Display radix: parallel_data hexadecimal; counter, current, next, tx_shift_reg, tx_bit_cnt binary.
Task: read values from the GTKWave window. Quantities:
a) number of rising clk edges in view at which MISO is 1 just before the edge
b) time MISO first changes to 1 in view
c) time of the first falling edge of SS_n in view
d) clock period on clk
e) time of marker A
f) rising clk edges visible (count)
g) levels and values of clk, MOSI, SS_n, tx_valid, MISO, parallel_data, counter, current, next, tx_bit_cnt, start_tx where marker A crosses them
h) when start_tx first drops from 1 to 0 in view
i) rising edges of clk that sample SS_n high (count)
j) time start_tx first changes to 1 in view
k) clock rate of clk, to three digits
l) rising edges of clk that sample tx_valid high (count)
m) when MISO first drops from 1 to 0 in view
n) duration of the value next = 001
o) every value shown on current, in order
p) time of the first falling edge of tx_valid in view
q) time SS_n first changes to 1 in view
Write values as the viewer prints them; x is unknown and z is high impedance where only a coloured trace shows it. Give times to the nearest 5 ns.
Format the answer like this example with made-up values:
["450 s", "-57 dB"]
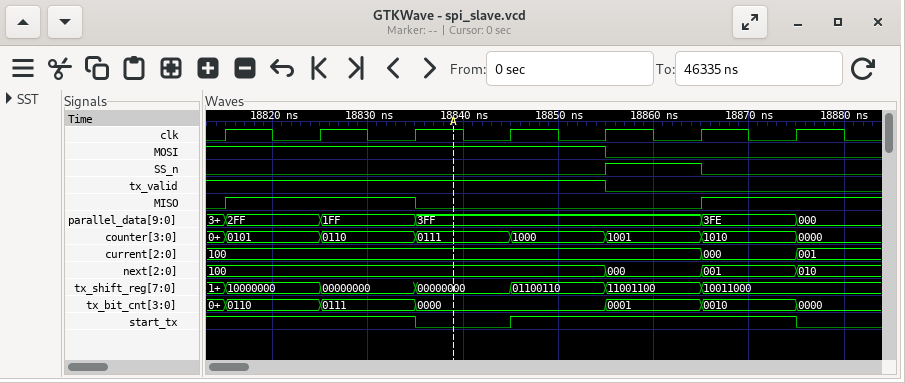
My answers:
["3", "18815 ns", "18865 ns", "10 ns", "18840 ns", "7", "clk=1, MOSI=1, SS_n=0, tx_valid=1, MISO=0, parallel_data=3FF, counter=0111, current=100, next=100, tx_bit_cnt=0000, start_tx=0", "18835 ns", "1", "18845 ns", "100 MHz", "5", "18835 ns", "10 ns", "100, 000, 001", "18855 ns", "18855 ns"]
